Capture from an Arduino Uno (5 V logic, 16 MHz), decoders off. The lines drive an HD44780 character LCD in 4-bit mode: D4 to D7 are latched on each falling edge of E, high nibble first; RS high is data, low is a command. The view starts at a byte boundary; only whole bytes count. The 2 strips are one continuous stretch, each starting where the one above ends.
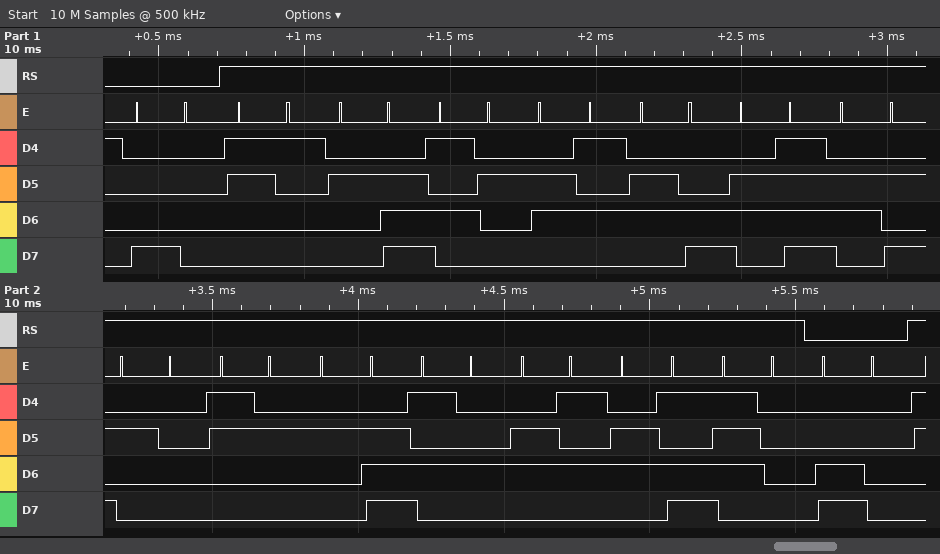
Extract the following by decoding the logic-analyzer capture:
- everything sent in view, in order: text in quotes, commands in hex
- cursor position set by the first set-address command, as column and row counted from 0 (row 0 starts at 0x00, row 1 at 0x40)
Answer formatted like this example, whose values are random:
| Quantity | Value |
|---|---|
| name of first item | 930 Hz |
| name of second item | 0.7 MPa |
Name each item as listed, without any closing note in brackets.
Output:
| Quantity | Value |
|---|---|
| everything sent in view, in order: text in quotes, commands in hex | 0x80 "1.Reloj 2.Temp" 0xC0 |
| cursor position set by the first set-address command, as column and row counted from 0 | column 0, row 0 |
